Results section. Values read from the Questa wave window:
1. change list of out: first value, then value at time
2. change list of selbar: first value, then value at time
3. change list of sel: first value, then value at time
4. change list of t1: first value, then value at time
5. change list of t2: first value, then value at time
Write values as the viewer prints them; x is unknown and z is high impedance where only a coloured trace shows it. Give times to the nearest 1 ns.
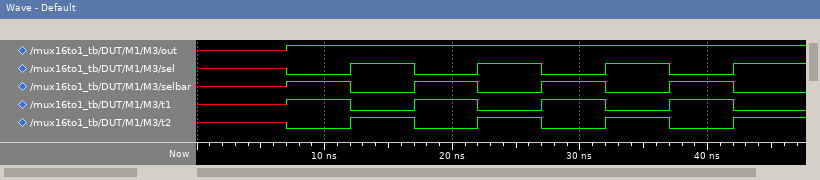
x, 1 at 7 ns
x, 1 at 7 ns, 0 at 12 ns, 1 at 17 ns, 0 at 22 ns, 1 at 27 ns, 0 at 32 ns, 1 at 37 ns, 0 at 42 ns
x, 0 at 7 ns, 1 at 12 ns, 0 at 17 ns, 1 at 22 ns, 0 at 27 ns, 1 at 32 ns, 0 at 37 ns, 1 at 42 ns
x, 1 at 7 ns, 0 at 12 ns, 1 at 17 ns, 0 at 22 ns, 1 at 27 ns, 0 at 32 ns, 1 at 37 ns, 0 at 42 ns
x, 0 at 7 ns, 1 at 12 ns, 0 at 17 ns, 1 at 22 ns, 0 at 27 ns, 1 at 32 ns, 0 at 37 ns, 1 at 42 ns
